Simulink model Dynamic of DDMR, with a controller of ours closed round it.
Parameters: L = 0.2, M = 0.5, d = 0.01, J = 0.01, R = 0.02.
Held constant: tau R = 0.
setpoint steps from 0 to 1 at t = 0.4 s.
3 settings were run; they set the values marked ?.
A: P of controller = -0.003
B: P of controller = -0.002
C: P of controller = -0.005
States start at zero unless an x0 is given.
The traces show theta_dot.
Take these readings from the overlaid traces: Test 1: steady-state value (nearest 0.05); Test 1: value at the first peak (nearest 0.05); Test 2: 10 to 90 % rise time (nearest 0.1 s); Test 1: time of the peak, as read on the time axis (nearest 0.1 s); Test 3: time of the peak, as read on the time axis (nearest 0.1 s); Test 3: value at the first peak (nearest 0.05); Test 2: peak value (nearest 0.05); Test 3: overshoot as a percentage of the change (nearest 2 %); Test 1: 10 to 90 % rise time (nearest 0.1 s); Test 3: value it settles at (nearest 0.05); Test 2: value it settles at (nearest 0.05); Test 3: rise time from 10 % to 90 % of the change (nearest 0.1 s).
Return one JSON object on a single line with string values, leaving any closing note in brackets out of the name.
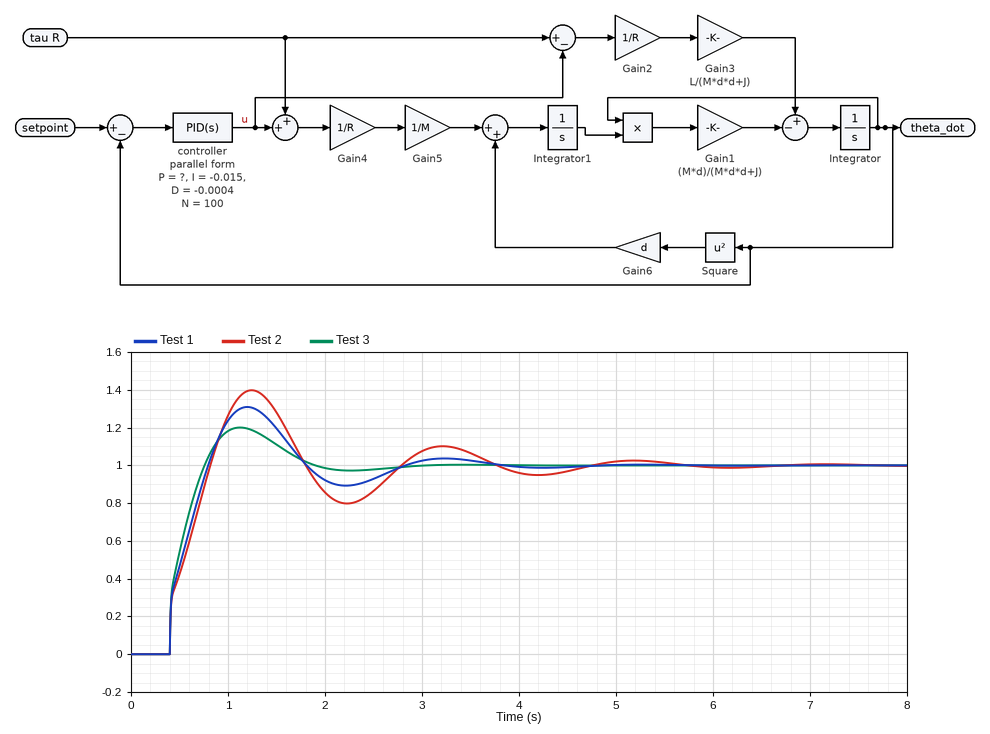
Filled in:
{"Test 1: steady-state value": "1.00", "Test 1: value at the first peak": "1.30", "Test 2: 10 to 90 % rise time": "0.4 s", "Test 1: time of the peak, as read on the time axis": "1.2 s", "Test 3: time of the peak, as read on the time axis": "1.1 s", "Test 3: value at the first peak": "1.20", "Test 2: peak value": "1.40", "Test 3: overshoot as a percentage of the change": "20 %", "Test 1: 10 to 90 % rise time": "0.3 s", "Test 3: value it settles at": "1.00", "Test 2: value it settles at": "1.00", "Test 3: rise time from 10 % to 90 % of the change": "0.3 s"}
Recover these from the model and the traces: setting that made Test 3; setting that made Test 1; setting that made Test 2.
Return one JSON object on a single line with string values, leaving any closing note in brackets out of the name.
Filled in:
{"setting that made Test 3": "C", "setting that made Test 1": "A", "setting that made Test 2": "B"}
